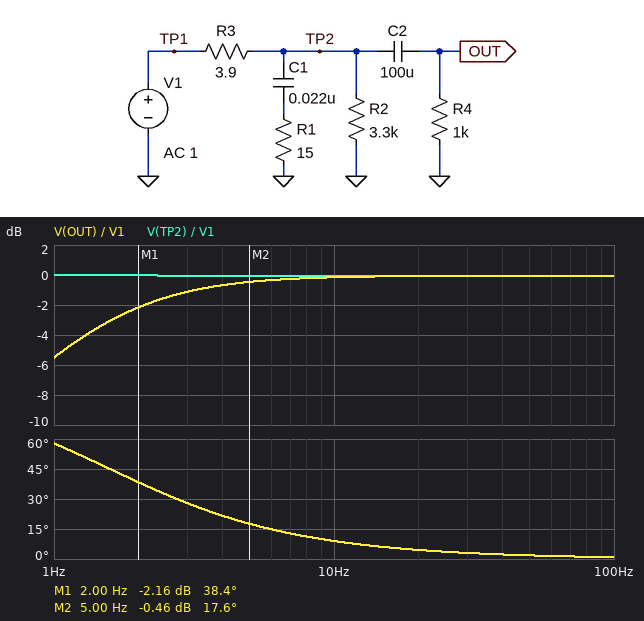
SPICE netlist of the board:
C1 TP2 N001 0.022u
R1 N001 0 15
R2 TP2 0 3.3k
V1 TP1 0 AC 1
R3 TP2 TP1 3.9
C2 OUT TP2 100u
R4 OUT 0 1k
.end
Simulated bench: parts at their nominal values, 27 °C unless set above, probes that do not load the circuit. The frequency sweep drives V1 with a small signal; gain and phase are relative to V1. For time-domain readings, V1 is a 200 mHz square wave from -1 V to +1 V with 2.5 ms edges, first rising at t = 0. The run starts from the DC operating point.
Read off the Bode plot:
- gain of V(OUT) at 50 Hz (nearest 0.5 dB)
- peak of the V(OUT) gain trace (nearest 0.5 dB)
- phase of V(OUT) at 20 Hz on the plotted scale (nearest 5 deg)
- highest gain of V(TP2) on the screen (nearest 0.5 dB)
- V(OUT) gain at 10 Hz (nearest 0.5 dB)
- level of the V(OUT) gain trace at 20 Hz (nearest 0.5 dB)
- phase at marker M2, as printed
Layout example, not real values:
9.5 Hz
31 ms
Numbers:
0 dB
0 dB
5 deg
0 dB
0 dB
0 dB
17.6 deg
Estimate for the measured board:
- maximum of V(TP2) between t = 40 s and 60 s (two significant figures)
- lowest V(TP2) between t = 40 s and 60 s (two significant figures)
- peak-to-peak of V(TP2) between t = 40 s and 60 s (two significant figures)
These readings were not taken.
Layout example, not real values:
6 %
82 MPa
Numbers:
1.0 V
-1.0 V
2.0 V
